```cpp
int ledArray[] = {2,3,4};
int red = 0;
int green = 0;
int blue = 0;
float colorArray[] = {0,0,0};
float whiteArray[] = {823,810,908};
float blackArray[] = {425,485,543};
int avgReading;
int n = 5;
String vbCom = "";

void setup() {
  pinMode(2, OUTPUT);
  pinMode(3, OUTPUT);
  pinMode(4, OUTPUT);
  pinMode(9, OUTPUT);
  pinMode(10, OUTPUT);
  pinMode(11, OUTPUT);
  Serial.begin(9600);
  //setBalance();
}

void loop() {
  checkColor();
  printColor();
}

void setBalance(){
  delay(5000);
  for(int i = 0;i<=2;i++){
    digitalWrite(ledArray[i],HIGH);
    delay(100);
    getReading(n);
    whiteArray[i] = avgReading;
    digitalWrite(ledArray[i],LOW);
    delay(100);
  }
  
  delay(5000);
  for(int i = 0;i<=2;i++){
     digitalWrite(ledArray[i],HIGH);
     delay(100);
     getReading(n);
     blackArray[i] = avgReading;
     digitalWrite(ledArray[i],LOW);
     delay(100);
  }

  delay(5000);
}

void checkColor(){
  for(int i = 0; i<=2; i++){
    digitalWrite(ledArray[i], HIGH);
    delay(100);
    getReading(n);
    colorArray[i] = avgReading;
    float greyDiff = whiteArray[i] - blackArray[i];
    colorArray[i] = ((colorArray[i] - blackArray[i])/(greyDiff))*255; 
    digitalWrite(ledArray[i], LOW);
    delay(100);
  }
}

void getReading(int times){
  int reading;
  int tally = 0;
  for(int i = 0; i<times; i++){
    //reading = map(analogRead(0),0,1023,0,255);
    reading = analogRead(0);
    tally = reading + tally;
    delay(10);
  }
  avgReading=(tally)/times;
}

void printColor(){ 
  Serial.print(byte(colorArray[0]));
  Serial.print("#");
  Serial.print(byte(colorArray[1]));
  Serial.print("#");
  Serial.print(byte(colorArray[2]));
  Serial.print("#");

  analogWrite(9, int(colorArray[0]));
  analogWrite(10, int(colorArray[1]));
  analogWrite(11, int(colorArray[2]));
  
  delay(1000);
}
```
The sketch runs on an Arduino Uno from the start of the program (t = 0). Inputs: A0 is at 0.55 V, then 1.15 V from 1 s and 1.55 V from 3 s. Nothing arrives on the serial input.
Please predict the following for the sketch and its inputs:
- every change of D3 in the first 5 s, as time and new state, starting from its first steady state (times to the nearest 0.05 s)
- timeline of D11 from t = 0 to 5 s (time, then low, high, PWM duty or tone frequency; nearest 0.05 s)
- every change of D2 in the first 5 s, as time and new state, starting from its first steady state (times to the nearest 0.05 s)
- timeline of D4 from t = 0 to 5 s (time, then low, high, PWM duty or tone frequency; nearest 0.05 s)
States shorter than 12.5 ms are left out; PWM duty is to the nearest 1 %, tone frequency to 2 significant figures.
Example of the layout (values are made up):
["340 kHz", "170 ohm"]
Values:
["0 s low; 0.25 s high; 0.4 s low; 2 s high; 2.15 s low; 3.75 s high; 3.9 s low", "0 s low; 0.75 s PWM 83 %; 2.5 s PWM 16 %; 4.25 s PWM 39 %", "0 s high; 0.15 s low; 1.75 s high; 1.9 s low; 3.5 s high; 3.65 s low", "0 s low; 0.5 s high; 0.65 s low; 2.25 s high; 2.4 s low; 4 s high; 4.15 s low"]
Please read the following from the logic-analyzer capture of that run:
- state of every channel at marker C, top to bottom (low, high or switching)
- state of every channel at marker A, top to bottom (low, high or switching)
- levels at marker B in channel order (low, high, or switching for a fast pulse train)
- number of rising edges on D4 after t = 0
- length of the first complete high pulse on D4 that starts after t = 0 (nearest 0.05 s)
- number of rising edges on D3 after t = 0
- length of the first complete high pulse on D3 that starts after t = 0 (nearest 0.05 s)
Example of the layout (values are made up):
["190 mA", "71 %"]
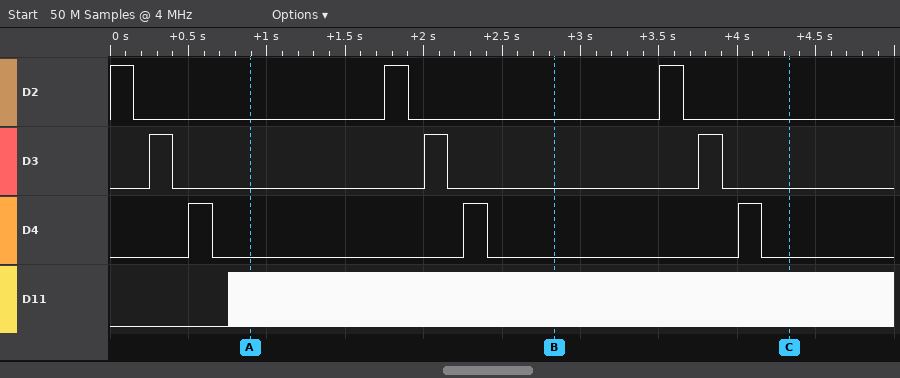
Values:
["D2 low, D3 low, D4 low, D11 switching", "D2 low, D3 low, D4 low, D11 switching", "D2 low, D3 low, D4 low, D11 switching", "3", "0.15 s", "3", "0.15 s"]
